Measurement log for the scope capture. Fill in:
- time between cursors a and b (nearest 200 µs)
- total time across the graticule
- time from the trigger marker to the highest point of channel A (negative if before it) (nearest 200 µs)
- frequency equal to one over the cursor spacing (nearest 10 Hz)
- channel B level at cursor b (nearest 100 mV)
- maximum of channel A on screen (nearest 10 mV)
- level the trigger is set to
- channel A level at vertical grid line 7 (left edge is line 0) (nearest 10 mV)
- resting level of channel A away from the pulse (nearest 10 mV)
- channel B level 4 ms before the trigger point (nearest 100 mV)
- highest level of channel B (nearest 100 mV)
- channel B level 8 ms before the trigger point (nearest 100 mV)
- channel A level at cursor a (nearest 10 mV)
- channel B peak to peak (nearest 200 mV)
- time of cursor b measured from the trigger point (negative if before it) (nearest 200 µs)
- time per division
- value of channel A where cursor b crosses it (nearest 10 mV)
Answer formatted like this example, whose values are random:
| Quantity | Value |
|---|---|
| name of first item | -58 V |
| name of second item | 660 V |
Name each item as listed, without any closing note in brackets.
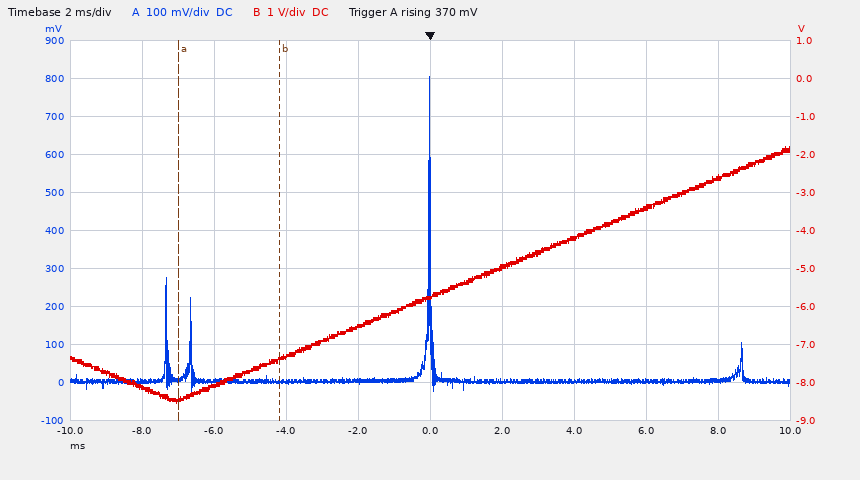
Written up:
| Quantity | Value |
|---|---|
| time between cursors a and b | 2.8 ms |
| total time across the graticule | 20 ms |
| time from the trigger marker to the highest point of channel A (negative if before it) | 0.0 ms |
| frequency equal to one over the cursor spacing | 360 Hz |
| channel B level at cursor b | -7.4 V |
| maximum of channel A on screen | 810 mV |
| level the trigger is set to | 370 mV |
| channel A level at vertical grid line 7 (left edge is line 0) | 0 mV |
| resting level of channel A away from the pulse | 0 mV |
| channel B level 4 ms before the trigger point | -7.3 V |
| highest level of channel B | -1.8 V |
| channel B level 8 ms before the trigger point | -8.1 V |
| channel A level at cursor a | 10 mV |
| channel B peak to peak | 6.8 V |
| time of cursor b measured from the trigger point (negative if before it) | -4.2 ms |
| time per division | 2 ms |
| value of channel A where cursor b crosses it | 0 mV |
